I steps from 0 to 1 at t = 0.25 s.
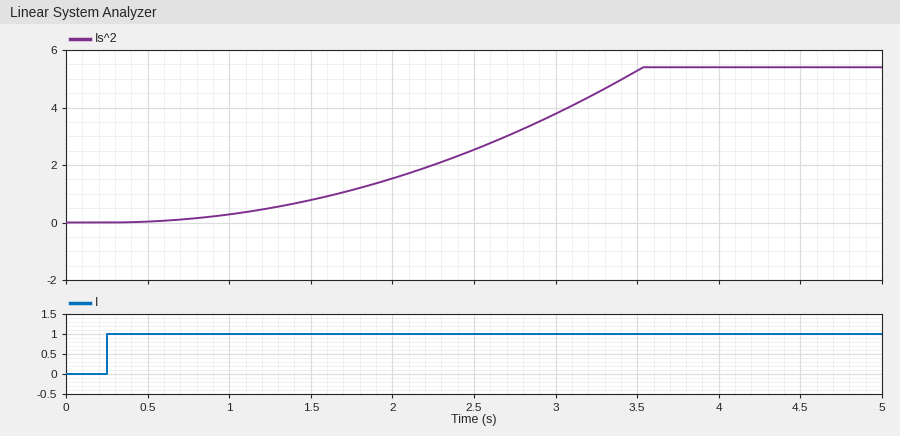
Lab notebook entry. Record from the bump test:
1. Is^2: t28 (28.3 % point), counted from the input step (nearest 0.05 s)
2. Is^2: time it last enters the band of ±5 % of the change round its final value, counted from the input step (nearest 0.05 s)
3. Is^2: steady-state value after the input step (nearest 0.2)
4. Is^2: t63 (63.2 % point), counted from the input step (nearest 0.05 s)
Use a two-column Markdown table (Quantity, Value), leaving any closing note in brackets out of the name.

| Quantity | Value |
|---|---|
| Is^2: t28 (28.3 % point), counted from the input step | 1.75 s |
| Is^2: time it last enters the band of ±5 % of the change round its final value, counted from the input step | 3.20 s |
| Is^2: steady-state value after the input step | 5.4 |
| Is^2: t63 (63.2 % point), counted from the input step | 2.60 s |
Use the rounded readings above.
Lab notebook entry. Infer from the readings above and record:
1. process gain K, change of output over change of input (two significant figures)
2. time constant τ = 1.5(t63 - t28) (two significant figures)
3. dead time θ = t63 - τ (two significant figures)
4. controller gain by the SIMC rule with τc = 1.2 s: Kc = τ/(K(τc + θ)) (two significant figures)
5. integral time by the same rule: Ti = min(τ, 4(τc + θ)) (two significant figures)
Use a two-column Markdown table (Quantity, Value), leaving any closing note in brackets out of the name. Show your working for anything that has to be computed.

| Quantity | Value |
|---|---|
| process gain K, change of output over change of input | (5.4 - 0) / 1 = 5.4 |
| time constant τ = 1.5(t63 - t28) | 1.5 × (2.6 - 1.75) = 1.3 s |
| dead time θ = t63 - τ | 2.6 - 1.3 = 1.3 s |
| controller gain by the SIMC rule with τc = 1.2 s: Kc = τ/(K(τc + θ)) | 1.3 / (5.4 × (1.2 + 1.3)) = 0.096 |
| integral time by the same rule: Ti = min(τ, 4(τc + θ)) | min(1.3, 4 × (1.2 + 1.3)) = 1.3 s |
